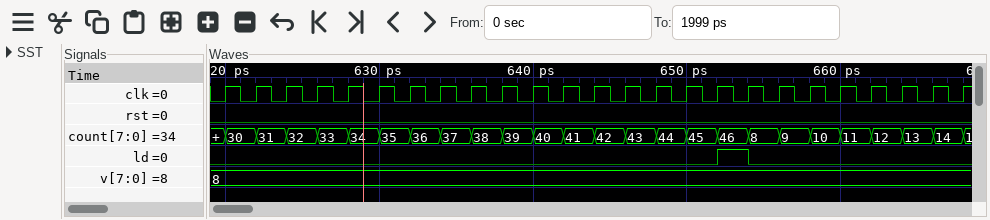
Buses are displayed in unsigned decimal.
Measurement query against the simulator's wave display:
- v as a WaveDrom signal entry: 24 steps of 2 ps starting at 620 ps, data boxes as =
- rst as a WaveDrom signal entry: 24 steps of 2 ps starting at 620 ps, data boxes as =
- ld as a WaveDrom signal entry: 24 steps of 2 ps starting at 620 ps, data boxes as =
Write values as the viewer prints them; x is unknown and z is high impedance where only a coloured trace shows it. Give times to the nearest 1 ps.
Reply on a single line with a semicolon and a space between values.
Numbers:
{name: 'v', wave: '=.......................', data: '8'}; {name: 'rst', wave: '0.......................'}; {name: 'ld', wave: '0...............10......'}
